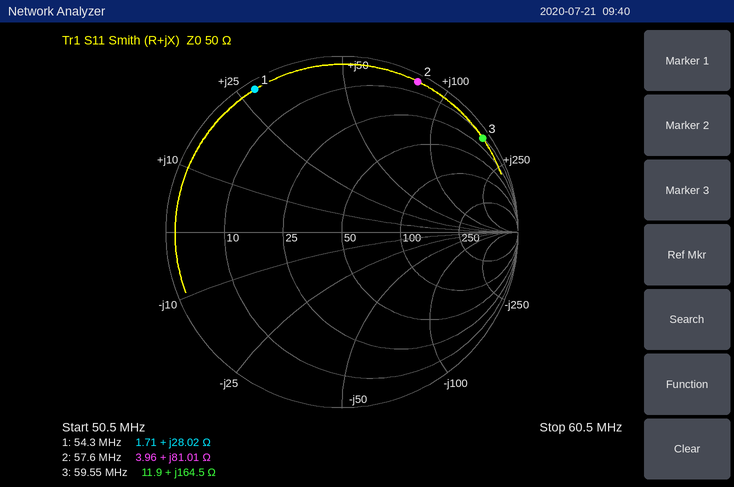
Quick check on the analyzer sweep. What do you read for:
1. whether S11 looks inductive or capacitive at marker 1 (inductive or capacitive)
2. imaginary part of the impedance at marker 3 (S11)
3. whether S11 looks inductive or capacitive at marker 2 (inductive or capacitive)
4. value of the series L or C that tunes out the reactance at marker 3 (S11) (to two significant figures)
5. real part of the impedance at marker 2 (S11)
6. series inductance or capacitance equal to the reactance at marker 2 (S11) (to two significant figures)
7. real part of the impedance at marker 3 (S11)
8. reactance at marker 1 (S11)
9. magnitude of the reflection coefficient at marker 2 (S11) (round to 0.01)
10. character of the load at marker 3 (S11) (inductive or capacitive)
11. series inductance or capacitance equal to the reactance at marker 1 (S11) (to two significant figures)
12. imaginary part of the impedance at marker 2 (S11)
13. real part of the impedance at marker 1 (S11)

inductive
+164.5 Ω
inductive
16 pF
3.96 Ω
220 nH
11.9 Ω
+28.02 Ω
0.96
inductive
82 nH
+81.01 Ω
1.71 Ω
